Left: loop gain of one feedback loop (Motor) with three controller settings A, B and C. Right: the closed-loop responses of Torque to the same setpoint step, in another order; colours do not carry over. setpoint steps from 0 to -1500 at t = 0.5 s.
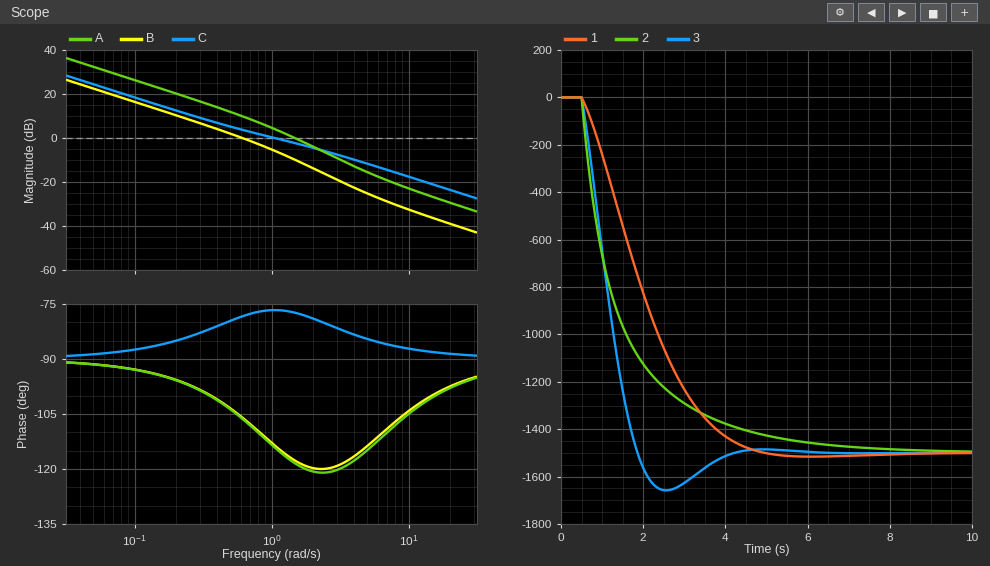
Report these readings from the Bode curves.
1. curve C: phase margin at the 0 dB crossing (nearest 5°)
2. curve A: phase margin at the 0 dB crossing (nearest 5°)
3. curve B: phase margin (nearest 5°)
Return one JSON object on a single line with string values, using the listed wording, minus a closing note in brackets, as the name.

{"curve C: phase margin at the 0 dB crossing": "105°", "curve A: phase margin at the 0 dB crossing": "60°", "curve B: phase margin": "75°"}
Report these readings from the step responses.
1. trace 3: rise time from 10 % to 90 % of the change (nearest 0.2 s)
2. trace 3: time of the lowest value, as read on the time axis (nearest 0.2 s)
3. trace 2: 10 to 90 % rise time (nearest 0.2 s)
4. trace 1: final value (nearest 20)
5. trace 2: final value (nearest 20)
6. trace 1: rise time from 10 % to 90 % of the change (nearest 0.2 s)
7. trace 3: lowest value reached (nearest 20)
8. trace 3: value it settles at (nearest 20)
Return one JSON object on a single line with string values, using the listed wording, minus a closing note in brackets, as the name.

{"trace 3: rise time from 10 % to 90 % of the change": "1.0 s", "trace 3: time of the lowest value, as read on the time axis": "2.6 s", "trace 2: 10 to 90 % rise time": "3.0 s", "trace 1: final value": "-1500", "trace 2: final value": "-1500", "trace 1: rise time from 10 % to 90 % of the change": "2.6 s", "trace 3: lowest value reached": "-1660", "trace 3: value it settles at": "-1500"}
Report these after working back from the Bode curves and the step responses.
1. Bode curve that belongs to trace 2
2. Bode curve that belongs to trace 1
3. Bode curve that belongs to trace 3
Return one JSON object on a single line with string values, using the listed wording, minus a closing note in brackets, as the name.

{"Bode curve that belongs to trace 2": "C", "Bode curve that belongs to trace 1": "B", "Bode curve that belongs to trace 3": "A"}
